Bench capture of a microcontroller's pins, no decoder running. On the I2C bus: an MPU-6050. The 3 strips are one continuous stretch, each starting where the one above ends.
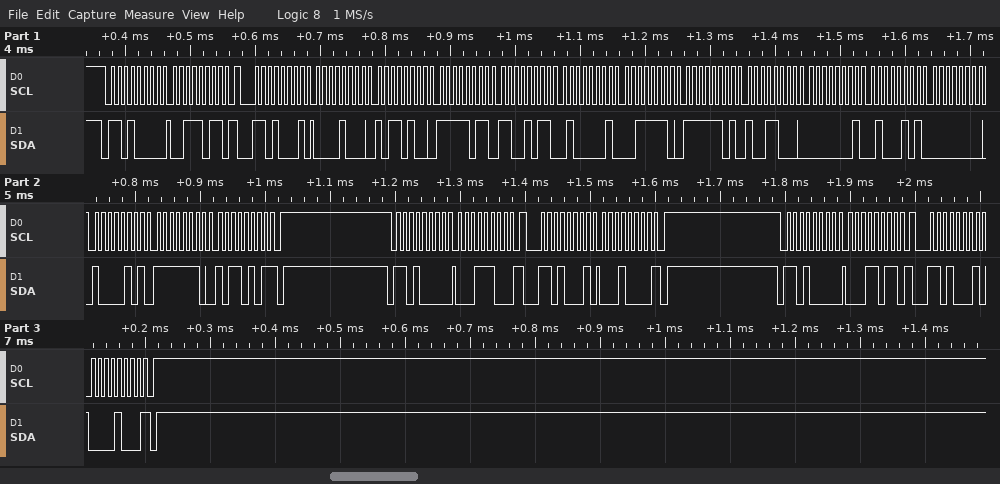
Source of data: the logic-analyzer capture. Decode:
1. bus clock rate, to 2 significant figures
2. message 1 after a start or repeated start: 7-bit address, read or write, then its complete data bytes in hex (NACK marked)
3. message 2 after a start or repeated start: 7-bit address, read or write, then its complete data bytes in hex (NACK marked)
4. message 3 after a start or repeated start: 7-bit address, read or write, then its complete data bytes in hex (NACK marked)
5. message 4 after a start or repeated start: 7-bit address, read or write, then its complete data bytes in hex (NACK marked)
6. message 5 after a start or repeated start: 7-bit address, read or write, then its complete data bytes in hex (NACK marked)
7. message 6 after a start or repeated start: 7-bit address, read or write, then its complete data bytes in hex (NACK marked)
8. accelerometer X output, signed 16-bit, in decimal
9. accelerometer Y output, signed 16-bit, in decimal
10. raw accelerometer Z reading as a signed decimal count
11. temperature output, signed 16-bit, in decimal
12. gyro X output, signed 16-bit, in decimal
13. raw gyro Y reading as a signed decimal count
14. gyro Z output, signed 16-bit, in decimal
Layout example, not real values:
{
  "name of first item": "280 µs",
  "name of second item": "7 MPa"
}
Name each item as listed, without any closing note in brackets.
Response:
{
  "bus clock rate, to 2 significant figures": "100 kHz",
  "message 1 after a start or repeated start: 7-bit address, read or write, then its complete data bytes in hex": "0x68 write: 3B",
  "message 2 after a start or repeated start: 7-bit address, read or write, then its complete data bytes in hex": "0x68 read: 08 B4 FB CB 41 3E FD 98 01 45 00 85 FE B5 NACK",
  "message 3 after a start or repeated start: 7-bit address, read or write, then its complete data bytes in hex": "0x68 write: 1C",
  "message 4 after a start or repeated start: 7-bit address, read or write, then its complete data bytes in hex": "0x68 read: 10 NACK",
  "message 5 after a start or repeated start: 7-bit address, read or write, then its complete data bytes in hex": "0x68 write: 1B",
  "message 6 after a start or repeated start: 7-bit address, read or write, then its complete data bytes in hex": "0x68 read: 08 NACK",
  "accelerometer X output, signed 16-bit, in decimal": "2228",
  "accelerometer Y output, signed 16-bit, in decimal": "-1077",
  "raw accelerometer Z reading as a signed decimal count": "16702",
  "temperature output, signed 16-bit, in decimal": "-616",
  "gyro X output, signed 16-bit, in decimal": "325",
  "raw gyro Y reading as a signed decimal count": "133",
  "gyro Z output, signed 16-bit, in decimal": "-331"
}
